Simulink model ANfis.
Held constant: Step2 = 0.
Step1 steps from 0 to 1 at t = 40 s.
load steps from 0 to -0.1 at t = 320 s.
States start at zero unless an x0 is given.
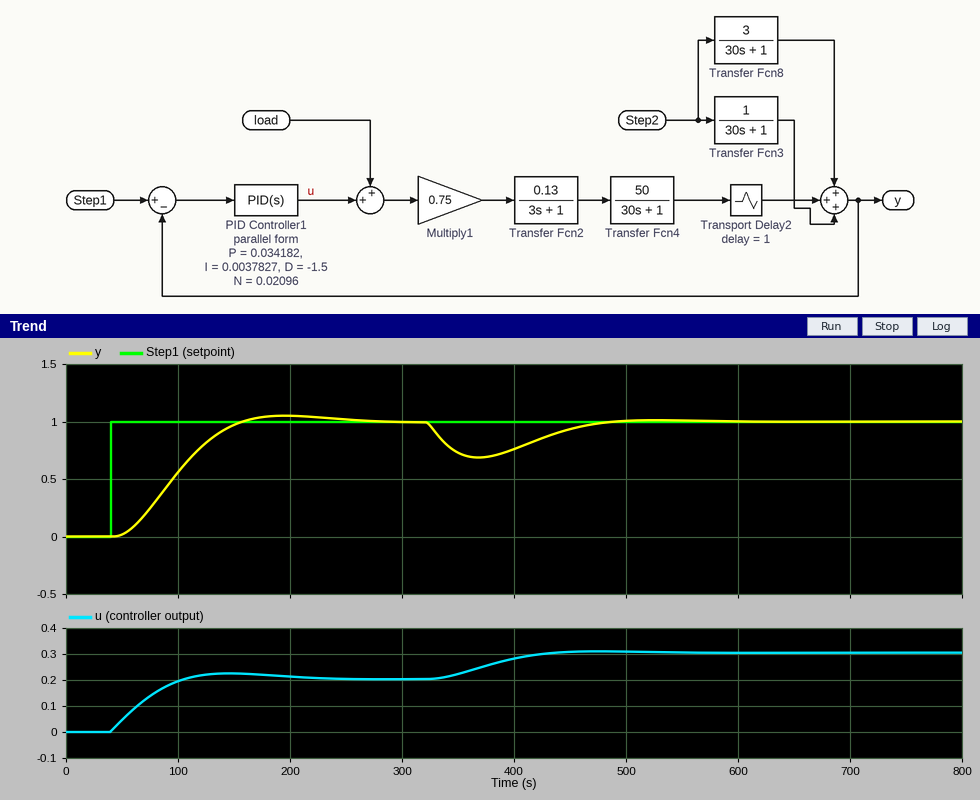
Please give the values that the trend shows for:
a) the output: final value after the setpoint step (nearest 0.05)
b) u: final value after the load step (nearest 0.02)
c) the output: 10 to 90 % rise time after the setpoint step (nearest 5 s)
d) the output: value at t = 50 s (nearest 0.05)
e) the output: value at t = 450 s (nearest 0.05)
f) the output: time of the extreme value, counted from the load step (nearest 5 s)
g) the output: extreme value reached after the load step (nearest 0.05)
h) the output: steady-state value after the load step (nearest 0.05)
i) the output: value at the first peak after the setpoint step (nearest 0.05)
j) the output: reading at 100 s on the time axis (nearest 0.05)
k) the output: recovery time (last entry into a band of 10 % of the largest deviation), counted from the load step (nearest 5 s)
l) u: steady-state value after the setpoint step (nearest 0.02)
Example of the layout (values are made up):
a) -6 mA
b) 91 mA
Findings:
a) 1.00
b) 0.30
c) 75 s
d) 0.00
e) 0.95
f) 50 s
g) 0.70
h) 1.00
i) 1.05
j) 0.55
k) 145 s
l) 0.20
